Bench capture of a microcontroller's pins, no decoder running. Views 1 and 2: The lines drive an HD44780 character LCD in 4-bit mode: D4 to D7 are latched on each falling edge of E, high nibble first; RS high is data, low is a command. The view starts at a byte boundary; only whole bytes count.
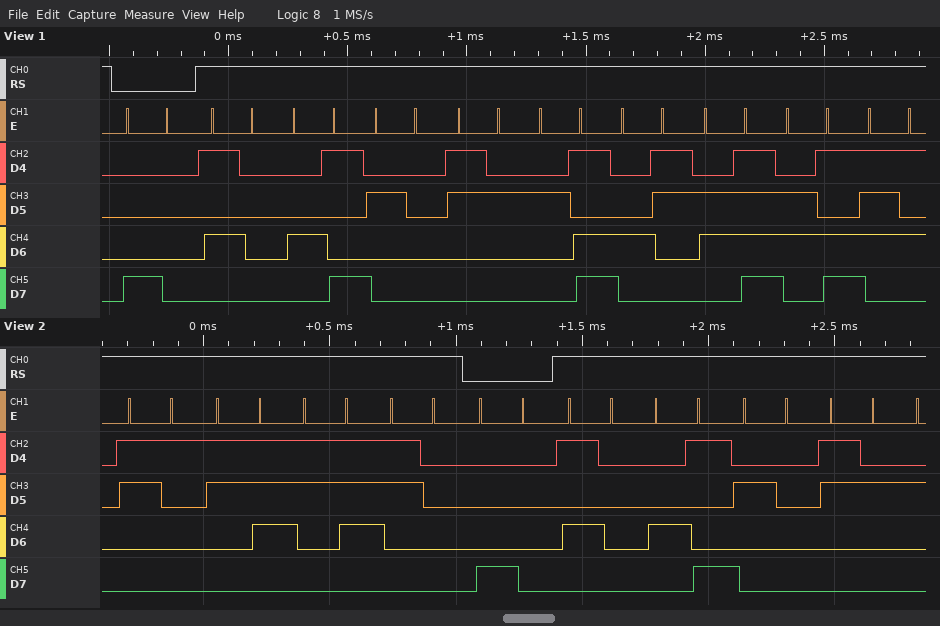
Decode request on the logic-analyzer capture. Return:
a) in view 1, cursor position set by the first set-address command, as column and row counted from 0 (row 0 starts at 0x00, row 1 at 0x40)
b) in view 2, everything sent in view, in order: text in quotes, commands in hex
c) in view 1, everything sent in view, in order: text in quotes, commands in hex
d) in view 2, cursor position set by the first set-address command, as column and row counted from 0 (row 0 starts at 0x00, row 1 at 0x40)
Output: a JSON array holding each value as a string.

["column 0, row 0", "\"1770\" 0x80 \"PI 2\"", "0x80 \"PI 2-Comu\"", "column 0, row 0"]
